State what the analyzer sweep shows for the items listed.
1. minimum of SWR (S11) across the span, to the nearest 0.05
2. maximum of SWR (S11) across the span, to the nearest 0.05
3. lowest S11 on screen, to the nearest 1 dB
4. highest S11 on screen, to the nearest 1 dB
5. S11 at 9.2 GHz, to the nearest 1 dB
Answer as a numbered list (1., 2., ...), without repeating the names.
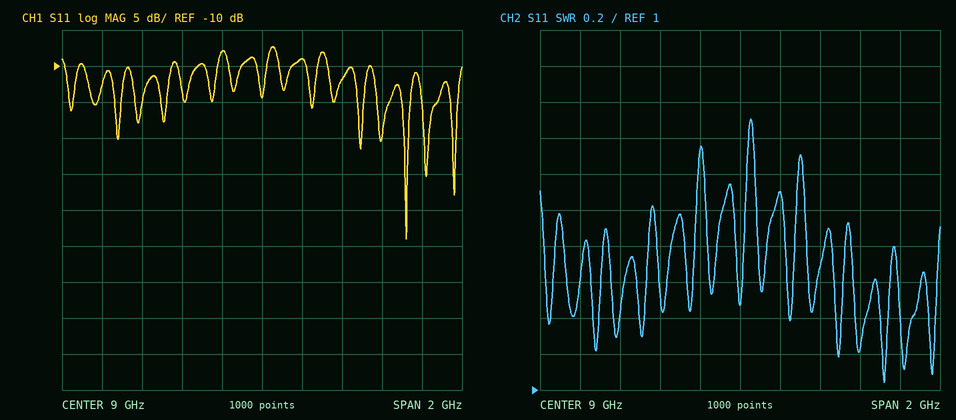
1. 1.05
2. 2.50
3. -34 dB
4. -7 dB
5. -9 dB
